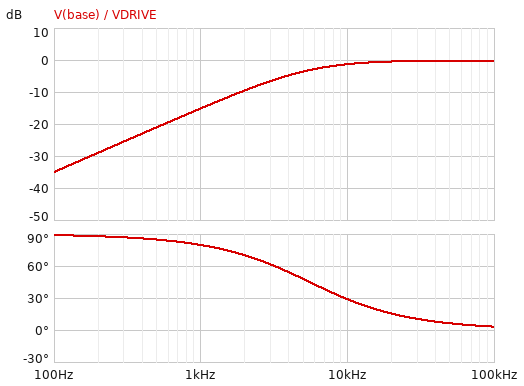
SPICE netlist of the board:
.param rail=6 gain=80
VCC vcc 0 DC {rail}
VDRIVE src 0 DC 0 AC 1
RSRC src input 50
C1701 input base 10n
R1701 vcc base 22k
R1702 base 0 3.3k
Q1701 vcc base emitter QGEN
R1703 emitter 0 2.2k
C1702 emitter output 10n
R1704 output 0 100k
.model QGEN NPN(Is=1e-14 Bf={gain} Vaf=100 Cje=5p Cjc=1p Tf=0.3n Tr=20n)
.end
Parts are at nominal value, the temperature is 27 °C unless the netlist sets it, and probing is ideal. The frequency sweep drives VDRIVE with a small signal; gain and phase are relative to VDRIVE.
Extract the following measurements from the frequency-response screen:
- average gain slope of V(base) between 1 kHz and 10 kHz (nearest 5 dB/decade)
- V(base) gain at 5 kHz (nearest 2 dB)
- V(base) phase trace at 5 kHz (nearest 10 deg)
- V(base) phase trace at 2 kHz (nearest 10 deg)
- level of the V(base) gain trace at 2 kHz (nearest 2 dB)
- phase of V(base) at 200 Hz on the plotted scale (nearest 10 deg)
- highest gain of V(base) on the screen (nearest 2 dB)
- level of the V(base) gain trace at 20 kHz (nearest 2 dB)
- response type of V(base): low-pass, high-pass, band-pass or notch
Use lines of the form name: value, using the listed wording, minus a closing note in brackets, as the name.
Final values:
average gain slope of V(base) between 1 kHz and 10 kHz: 15 dB/decade
V(base) gain at 5 kHz: -4 dB
V(base) phase trace at 5 kHz: 50 deg
V(base) phase trace at 2 kHz: 70 deg
level of the V(base) gain trace at 2 kHz: -10 dB
phase of V(base) at 200 Hz on the plotted scale: 90 deg
highest gain of V(base) on the screen: 0 dB
level of the V(base) gain trace at 20 kHz: 0 dB
response type of V(base): low-pass, high-pass, band-pass or notch: high-pass
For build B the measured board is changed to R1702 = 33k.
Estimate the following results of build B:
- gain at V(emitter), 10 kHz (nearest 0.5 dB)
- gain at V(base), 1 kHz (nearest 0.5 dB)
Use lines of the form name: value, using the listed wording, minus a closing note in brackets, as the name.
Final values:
gain at V(emitter), 10 kHz: 0 dB
gain at V(base), 1 kHz: -4.5 dB
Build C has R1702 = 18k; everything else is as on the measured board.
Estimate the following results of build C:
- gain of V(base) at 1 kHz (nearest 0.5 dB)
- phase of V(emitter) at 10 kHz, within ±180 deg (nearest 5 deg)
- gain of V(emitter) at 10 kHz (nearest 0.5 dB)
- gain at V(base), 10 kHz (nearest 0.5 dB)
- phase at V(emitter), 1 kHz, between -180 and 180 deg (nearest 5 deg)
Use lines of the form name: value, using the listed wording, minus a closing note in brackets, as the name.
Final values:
gain of V(base) at 1 kHz: -6.0 dB
phase of V(emitter) at 10 kHz, within ±180 deg: 10 deg
gain of V(emitter) at 10 kHz: -0.5 dB
gain at V(base), 10 kHz: 0 dB
phase at V(emitter), 1 kHz, between -180 and 180 deg: 60 deg
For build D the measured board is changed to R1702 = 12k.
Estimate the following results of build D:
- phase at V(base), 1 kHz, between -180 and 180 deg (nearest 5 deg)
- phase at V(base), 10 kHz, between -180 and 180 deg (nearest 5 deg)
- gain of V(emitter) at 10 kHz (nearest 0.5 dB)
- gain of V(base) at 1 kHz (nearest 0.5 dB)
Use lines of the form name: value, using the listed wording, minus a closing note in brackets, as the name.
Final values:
phase at V(base), 1 kHz, between -180 and 180 deg: 65 deg
phase at V(base), 10 kHz, between -180 and 180 deg: 10 deg
gain of V(emitter) at 10 kHz: -0.5 dB
gain of V(base) at 1 kHz: -7.5 dB
